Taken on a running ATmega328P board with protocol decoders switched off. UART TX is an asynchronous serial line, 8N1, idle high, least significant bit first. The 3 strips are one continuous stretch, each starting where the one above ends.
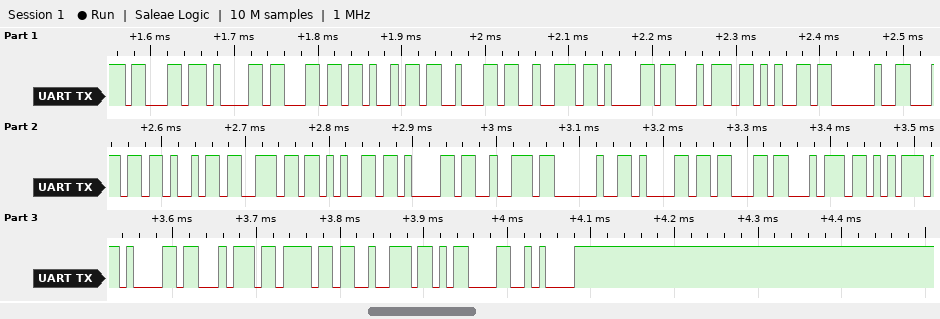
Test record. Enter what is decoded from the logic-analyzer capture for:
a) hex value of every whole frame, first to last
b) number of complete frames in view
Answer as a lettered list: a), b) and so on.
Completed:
a) 63 61 6C 69 62 72 61 74 65 20 6C 69 6E 65 61 72 20 61 63 74 75 61 74 6F 72 0D 0A
b) 27
